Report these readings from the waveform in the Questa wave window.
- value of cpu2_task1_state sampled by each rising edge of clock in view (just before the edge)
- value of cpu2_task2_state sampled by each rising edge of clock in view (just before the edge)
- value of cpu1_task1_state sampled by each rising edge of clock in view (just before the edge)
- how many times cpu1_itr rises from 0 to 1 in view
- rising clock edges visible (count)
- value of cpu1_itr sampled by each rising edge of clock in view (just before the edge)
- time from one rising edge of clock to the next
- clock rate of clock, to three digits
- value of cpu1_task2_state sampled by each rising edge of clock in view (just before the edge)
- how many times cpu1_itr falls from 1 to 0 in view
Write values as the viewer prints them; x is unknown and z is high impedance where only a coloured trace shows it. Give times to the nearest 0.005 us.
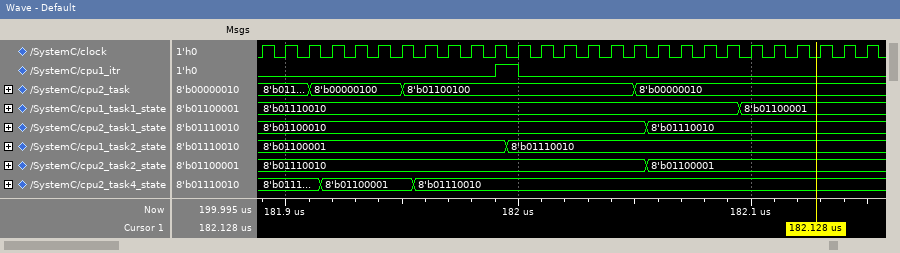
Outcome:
8'b01100010, 8'b01100010, 8'b01100010, 8'b01100010, 8'b01100010, 8'b01100010, 8'b01100010, 8'b01100010, 8'b01100010, 8'b01100010, 8'b01100010, 8'b01100010, 8'b01100010, 8'b01100010, 8'b01100010, 8'b01100010, 8'b01100010, 8'b01110010, 8'b01110010, 8'b01110010, 8'b01110010, 8'b01110010, 8'b01110010, 8'b01110010, 8'b01110010, 8'b01110010, 8'b01110010
8'b01110010, 8'b01110010, 8'b01110010, 8'b01110010, 8'b01110010, 8'b01110010, 8'b01110010, 8'b01110010, 8'b01110010, 8'b01110010, 8'b01110010, 8'b01110010, 8'b01110010, 8'b01110010, 8'b01110010, 8'b01110010, 8'b01110010, 8'b01100001, 8'b01100001, 8'b01100001, 8'b01100001, 8'b01100001, 8'b01100001, 8'b01100001, 8'b01100001, 8'b01100001, 8'b01100001
8'b01110010, 8'b01110010, 8'b01110010, 8'b01110010, 8'b01110010, 8'b01110010, 8'b01110010, 8'b01110010, 8'b01110010, 8'b01110010, 8'b01110010, 8'b01110010, 8'b01110010, 8'b01110010, 8'b01110010, 8'b01110010, 8'b01110010, 8'b01110010, 8'b01110010, 8'b01110010, 8'b01110010, 8'b01100001, 8'b01100001, 8'b01100001, 8'b01100001, 8'b01100001, 8'b01100001
1
27
0 0 0 0 0 0 0 0 0 0 0 1 0 0 0 0 0 0 0 0 0 0 0 0 0 0 0
0.01 us
100 MHz
8'b01100001, 8'b01100001, 8'b01100001, 8'b01100001, 8'b01100001, 8'b01100001, 8'b01100001, 8'b01100001, 8'b01100001, 8'b01100001, 8'b01100001, 8'b01110010, 8'b01110010, 8'b01110010, 8'b01110010, 8'b01110010, 8'b01110010, 8'b01110010, 8'b01110010, 8'b01110010, 8'b01110010, 8'b01110010, 8'b01110010, 8'b01110010, 8'b01110010, 8'b01110010, 8'b01110010
1
